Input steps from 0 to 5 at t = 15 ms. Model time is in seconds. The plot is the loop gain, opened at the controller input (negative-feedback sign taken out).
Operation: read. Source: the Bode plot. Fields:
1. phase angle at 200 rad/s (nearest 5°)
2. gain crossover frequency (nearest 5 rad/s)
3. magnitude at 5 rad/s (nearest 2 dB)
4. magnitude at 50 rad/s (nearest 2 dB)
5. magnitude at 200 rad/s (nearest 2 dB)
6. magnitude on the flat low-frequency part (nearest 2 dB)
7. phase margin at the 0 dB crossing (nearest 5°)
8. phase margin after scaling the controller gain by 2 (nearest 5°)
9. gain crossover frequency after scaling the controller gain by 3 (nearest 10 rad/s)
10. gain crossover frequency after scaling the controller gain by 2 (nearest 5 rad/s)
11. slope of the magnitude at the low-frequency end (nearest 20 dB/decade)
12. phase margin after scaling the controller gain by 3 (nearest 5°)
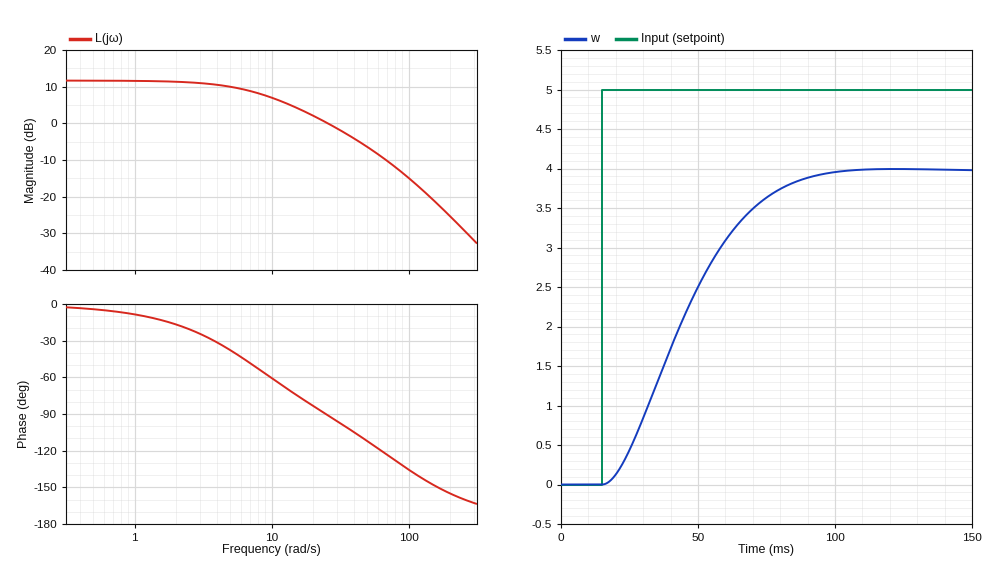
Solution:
-155°
25 rad/s
10 dB
-6 dB
-26 dB
12 dB
90°
70°
70 rad/s
50 rad/s
0 dB/decade
60°
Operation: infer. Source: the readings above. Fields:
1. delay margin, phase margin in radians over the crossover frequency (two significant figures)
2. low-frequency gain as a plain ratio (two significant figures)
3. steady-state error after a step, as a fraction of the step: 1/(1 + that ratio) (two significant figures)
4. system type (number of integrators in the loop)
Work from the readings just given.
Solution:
0.063 s
4.0
0.20
0
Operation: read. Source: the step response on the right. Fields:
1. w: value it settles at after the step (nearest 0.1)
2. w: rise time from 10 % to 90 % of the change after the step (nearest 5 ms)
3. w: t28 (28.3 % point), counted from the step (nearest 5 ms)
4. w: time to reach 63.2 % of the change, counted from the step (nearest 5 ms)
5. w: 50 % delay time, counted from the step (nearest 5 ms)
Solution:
4.0
50 ms
20 ms
35 ms
30 ms
